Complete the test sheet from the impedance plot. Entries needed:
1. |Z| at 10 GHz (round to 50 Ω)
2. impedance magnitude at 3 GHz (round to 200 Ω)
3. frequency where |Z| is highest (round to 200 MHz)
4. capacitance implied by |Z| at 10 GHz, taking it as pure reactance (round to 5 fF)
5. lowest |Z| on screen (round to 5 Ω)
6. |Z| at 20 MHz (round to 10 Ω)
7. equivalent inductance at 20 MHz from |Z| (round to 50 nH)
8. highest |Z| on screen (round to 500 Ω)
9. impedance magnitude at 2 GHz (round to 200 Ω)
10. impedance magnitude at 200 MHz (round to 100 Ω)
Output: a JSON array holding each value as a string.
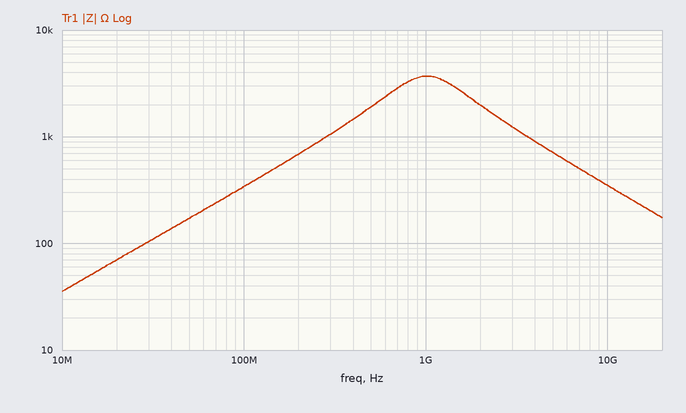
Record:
["350 Ω", "1.2 kΩ", "1.0 GHz", "45 fF", "35 Ω", "70 Ω", "550 nH", "3.5 kΩ", "2.0 kΩ", "700 Ω"]
